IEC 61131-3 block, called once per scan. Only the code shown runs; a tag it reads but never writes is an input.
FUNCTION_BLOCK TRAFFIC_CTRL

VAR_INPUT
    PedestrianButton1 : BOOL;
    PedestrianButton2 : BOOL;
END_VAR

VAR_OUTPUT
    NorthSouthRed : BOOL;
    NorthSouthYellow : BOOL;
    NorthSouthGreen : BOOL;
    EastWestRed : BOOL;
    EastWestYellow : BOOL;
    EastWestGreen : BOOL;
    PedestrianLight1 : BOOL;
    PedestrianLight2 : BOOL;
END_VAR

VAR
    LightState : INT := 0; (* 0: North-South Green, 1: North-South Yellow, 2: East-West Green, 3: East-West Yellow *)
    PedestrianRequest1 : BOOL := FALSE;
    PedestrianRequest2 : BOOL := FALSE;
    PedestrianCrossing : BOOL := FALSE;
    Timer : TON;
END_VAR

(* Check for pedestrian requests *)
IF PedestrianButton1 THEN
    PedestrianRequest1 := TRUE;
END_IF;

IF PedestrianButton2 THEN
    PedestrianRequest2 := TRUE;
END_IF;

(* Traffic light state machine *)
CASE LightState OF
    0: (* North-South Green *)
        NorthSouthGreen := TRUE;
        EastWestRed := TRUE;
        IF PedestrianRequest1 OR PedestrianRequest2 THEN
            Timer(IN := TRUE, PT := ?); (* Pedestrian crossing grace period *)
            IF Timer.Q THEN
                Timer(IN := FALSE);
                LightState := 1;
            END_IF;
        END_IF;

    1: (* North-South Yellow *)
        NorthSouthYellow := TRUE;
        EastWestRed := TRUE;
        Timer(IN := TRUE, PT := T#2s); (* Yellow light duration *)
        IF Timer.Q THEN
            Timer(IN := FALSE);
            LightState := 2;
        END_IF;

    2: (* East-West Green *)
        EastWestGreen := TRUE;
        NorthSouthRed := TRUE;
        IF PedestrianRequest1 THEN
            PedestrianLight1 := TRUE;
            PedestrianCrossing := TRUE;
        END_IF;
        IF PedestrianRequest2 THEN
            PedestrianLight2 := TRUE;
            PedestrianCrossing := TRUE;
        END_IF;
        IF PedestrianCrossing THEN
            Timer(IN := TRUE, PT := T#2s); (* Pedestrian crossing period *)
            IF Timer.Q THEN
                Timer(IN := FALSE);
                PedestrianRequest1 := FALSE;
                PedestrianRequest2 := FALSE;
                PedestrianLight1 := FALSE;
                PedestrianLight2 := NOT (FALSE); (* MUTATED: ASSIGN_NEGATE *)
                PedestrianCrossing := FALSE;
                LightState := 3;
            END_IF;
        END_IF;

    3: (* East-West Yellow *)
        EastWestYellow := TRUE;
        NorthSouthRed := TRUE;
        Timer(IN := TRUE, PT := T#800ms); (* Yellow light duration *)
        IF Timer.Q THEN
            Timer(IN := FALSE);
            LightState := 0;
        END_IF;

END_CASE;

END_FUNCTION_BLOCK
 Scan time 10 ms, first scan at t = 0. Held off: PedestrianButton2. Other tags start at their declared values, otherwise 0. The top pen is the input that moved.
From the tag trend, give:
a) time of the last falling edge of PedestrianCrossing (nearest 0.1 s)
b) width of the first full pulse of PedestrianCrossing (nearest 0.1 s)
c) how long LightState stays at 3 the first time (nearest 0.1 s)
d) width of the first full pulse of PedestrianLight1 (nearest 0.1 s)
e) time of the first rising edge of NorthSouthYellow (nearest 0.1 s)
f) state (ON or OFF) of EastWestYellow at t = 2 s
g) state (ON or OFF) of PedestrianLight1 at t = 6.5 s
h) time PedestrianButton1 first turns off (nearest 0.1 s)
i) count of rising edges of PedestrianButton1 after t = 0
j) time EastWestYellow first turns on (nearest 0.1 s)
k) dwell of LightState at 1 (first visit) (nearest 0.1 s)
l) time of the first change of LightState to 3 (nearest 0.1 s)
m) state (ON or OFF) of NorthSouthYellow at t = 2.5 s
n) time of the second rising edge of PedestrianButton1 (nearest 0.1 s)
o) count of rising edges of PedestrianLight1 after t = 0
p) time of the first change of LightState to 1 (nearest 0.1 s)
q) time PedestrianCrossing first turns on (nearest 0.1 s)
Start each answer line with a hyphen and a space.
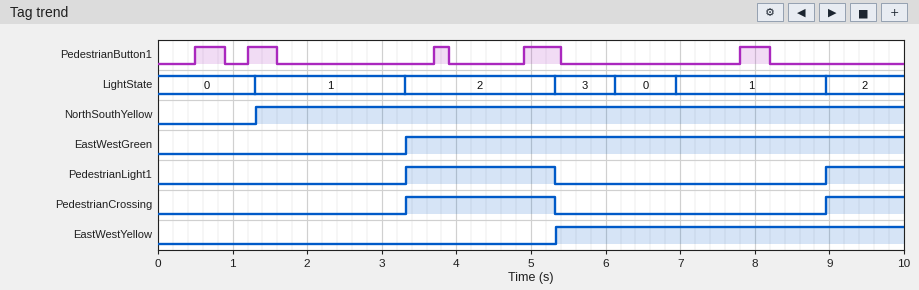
- 5.3 s
- 2.0 s
- 0.8 s
- 2.0 s
- 1.3 s
- OFF
- OFF
- 0.9 s
- 5
- 5.3 s
- 2.0 s
- 5.3 s
- ON
- 1.2 s
- 2
- 1.3 s
- 3.3 s
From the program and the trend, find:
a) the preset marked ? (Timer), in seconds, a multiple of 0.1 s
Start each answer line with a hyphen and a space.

- 0.8 s
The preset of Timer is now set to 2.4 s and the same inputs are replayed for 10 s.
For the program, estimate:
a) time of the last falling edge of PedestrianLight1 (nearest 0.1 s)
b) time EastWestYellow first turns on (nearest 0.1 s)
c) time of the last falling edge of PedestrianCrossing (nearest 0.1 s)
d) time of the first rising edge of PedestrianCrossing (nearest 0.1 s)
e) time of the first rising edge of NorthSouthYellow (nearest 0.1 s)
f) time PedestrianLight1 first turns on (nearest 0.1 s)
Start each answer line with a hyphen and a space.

- 6.9 s
- 6.9 s
- 6.9 s
- 4.9 s
- 2.9 s
- 4.9 s
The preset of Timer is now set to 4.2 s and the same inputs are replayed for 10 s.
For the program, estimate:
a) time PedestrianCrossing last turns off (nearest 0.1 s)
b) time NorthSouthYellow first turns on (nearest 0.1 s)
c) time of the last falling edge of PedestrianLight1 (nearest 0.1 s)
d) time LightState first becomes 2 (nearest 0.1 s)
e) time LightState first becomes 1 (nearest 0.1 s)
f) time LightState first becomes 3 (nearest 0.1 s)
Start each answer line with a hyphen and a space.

- 8.7 s
- 4.7 s
- 8.7 s
- 6.7 s
- 4.7 s
- 8.7 s
